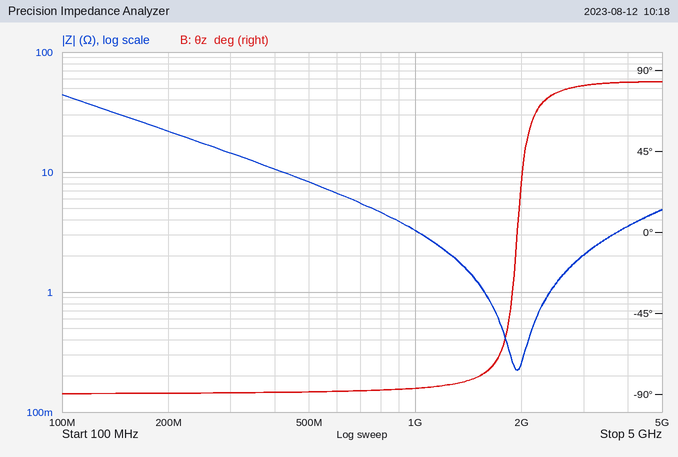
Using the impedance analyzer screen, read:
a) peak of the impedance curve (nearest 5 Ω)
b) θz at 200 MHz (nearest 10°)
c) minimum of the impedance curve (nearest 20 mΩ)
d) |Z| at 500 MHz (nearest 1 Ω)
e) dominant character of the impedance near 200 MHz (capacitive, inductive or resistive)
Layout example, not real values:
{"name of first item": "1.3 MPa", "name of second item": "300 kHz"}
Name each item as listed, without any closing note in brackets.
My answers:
{"peak of the impedance curve": "45 Ω", "θz at 200 MHz": "-90°", "minimum of the impedance curve": "220 mΩ", "|Z| at 500 MHz": "8 Ω", "dominant character of the impedance near 200 MHz": "capacitive"}
